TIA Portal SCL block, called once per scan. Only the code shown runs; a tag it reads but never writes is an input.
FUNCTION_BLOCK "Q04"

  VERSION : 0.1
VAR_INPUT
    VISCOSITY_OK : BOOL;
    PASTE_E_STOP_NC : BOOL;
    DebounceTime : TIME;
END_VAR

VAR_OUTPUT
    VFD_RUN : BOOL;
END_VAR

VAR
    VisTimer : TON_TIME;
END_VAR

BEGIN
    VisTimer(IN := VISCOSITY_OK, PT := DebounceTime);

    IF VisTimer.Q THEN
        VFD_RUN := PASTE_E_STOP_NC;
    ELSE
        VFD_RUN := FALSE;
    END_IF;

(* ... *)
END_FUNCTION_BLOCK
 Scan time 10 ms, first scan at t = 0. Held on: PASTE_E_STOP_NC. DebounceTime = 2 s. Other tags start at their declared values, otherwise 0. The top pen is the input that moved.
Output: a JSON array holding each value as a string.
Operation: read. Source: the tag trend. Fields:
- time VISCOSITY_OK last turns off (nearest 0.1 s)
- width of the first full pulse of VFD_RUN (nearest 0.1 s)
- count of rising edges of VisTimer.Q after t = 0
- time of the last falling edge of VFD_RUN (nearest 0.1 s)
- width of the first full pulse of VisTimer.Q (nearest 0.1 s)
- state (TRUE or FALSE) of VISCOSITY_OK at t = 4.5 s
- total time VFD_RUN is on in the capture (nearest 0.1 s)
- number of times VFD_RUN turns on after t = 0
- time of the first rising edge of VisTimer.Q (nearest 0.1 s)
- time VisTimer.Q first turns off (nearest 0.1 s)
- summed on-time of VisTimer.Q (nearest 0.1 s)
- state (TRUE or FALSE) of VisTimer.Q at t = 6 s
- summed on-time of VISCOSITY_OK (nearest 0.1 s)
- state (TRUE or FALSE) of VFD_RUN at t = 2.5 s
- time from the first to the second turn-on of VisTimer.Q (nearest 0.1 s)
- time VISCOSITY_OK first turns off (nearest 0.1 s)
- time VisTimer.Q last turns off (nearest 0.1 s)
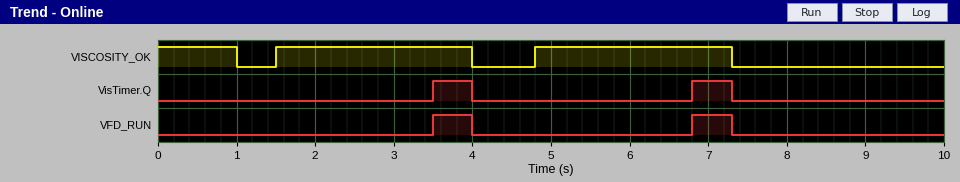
["7.3 s", "0.5 s", "2", "7.3 s", "0.5 s", "FALSE", "1.0 s", "2", "3.5 s", "4.0 s", "1.0 s", "FALSE", "6.0 s", "FALSE", "3.3 s", "1.0 s", "7.3 s"]
